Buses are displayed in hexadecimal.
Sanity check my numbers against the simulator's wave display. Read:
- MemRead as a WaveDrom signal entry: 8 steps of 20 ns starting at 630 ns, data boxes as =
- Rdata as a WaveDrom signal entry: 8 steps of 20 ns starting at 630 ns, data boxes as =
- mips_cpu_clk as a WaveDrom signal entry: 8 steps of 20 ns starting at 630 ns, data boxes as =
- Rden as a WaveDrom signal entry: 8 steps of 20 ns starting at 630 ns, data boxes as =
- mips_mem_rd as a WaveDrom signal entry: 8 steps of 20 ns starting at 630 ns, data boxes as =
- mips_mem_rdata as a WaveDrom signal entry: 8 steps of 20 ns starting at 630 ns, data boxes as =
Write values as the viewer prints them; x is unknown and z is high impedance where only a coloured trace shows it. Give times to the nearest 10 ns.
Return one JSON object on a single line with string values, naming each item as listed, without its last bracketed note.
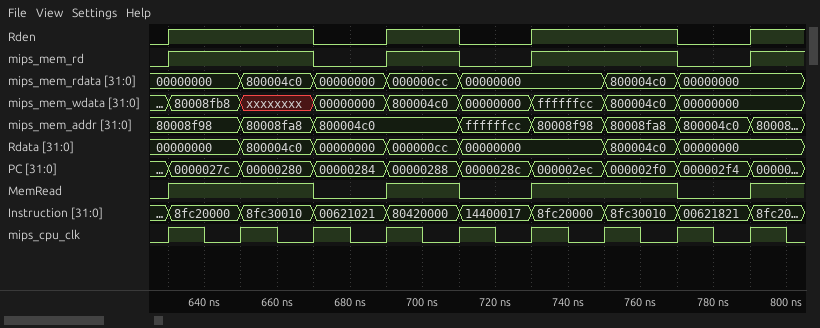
{"MemRead as a WaveDrom signal entry: 8 steps of 20 ns starting at 630 ns, data boxes as =": "{name: 'MemRead', wave: '1.0101.0'}", "Rdata as a WaveDrom signal entry: 8 steps of 20 ns starting at 630 ns, data boxes as =": "{name: 'Rdata', wave: '=====.==', data: '00000000 800004c0 00000000 000000cc 00000000 800004c0 00000000'}", "mips_cpu_clk as a WaveDrom signal entry: 8 steps of 20 ns starting at 630 ns, data boxes as =": "{name: 'mips_cpu_clk', wave: 'p.......'}", "Rden as a WaveDrom signal entry: 8 steps of 20 ns starting at 630 ns, data boxes as =": "{name: 'Rden', wave: '1.0101.0'}", "mips_mem_rd as a WaveDrom signal entry: 8 steps of 20 ns starting at 630 ns, data boxes as =": "{name: 'mips_mem_rd', wave: '1.0101.0'}", "mips_mem_rdata as a WaveDrom signal entry: 8 steps of 20 ns starting at 630 ns, data boxes as =": "{name: 'mips_mem_rdata', wave: '=====.==', data: '00000000 800004c0 00000000 000000cc 00000000 800004c0 00000000'}"}
